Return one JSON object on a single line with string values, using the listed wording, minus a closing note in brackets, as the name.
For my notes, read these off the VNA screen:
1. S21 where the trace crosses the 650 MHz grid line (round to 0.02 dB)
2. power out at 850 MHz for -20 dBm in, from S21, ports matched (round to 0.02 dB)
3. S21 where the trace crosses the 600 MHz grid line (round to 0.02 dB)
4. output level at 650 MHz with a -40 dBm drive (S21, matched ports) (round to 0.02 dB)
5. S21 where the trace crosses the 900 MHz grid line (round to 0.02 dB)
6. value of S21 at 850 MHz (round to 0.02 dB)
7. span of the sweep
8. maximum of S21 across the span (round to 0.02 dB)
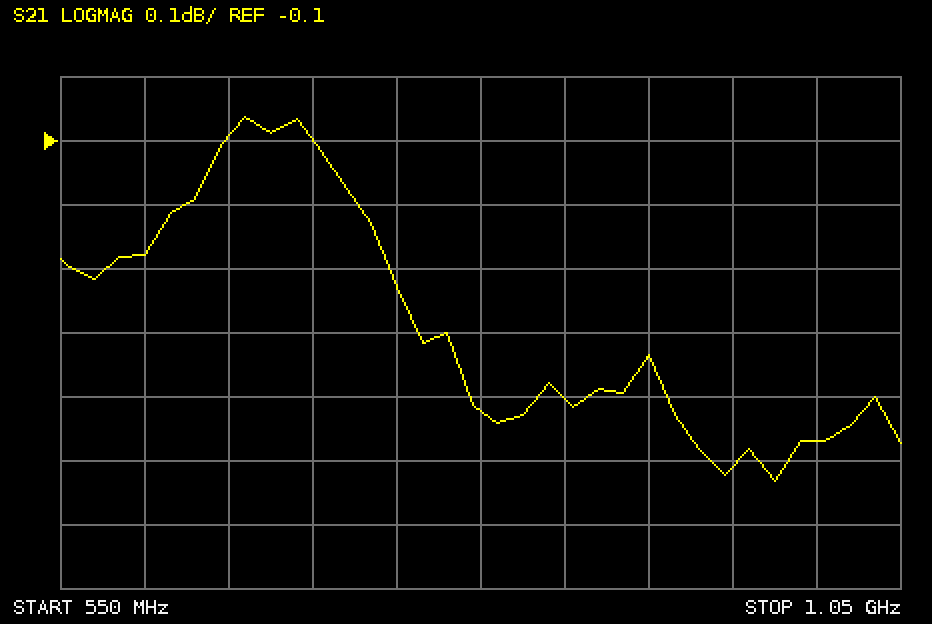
{"S21 where the trace crosses the 650 MHz grid line": "-0.10 dB", "power out at 850 MHz for -20 dBm in, from S21, ports matched": "-20.50 dBm", "S21 where the trace crosses the 600 MHz grid line": "-0.28 dB", "output level at 650 MHz with a -40 dBm drive (S21, matched ports)": "-40.10 dBm", "S21 where the trace crosses the 900 MHz grid line": "-0.44 dB", "value of S21 at 850 MHz": "-0.50 dB", "span of the sweep": "500 MHz", "maximum of S21 across the span": "-0.06 dB"}
